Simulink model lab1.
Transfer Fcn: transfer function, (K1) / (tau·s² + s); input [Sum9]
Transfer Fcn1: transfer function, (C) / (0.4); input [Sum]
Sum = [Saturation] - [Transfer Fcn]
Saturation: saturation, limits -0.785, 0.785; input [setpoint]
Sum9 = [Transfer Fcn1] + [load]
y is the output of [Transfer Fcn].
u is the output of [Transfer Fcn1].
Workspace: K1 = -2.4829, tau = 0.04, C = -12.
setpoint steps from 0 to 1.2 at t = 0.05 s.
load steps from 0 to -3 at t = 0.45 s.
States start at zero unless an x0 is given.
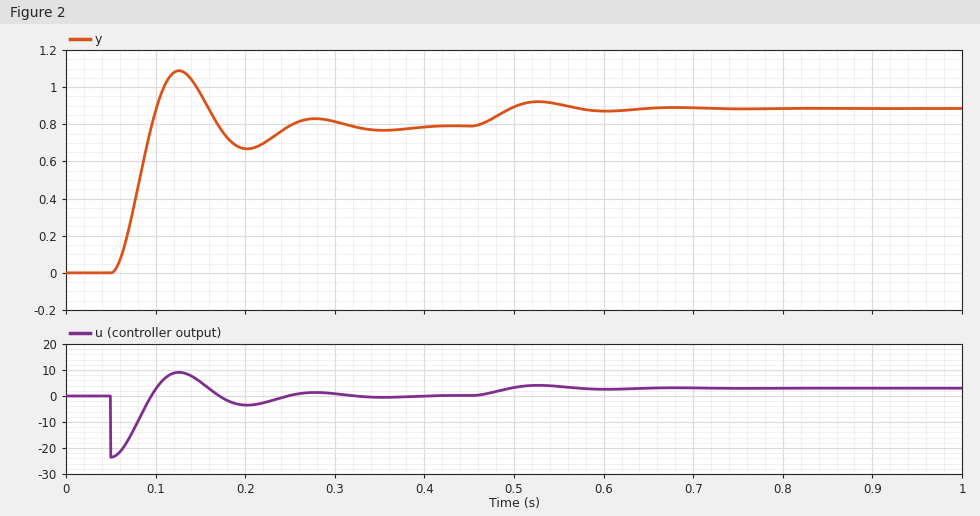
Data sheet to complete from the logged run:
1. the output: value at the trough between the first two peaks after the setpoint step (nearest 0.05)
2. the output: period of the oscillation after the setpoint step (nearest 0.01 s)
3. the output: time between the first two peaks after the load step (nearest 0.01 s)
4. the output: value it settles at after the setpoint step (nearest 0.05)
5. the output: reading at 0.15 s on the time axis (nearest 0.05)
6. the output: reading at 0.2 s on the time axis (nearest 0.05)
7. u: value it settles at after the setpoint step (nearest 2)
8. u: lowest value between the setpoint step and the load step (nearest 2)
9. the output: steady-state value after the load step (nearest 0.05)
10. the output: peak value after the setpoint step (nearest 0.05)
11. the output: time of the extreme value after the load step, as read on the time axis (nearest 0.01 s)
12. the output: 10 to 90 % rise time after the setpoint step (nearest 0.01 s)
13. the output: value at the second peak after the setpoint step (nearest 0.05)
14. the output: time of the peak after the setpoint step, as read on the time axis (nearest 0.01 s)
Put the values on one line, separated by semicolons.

0.65; 0.15 s; 0.15 s; 0.80; 0.95; 0.65; 0; -24; 0.90; 1.10; 0.53 s; 0.03 s; 0.85; 0.13 s
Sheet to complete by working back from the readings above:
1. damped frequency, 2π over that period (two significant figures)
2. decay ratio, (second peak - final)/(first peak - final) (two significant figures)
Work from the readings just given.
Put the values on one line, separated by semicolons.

42 rad/s; 0.17
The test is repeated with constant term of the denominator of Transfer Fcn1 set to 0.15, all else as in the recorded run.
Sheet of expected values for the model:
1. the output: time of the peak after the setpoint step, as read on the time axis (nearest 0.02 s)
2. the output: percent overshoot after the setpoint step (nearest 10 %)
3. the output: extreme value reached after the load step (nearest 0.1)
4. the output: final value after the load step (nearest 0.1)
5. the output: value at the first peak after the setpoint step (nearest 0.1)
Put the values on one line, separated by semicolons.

0.10 s; 60 %; 0.8; 0.8; 1.2
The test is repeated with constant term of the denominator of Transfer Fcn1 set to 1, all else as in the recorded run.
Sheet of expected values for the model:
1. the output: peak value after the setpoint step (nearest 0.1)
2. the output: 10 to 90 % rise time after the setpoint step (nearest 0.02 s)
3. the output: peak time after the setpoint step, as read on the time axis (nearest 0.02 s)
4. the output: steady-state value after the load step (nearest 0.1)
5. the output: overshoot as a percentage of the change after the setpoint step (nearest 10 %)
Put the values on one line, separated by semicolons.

0.9; 0.06 s; 0.18 s; 1.0; 20 %
